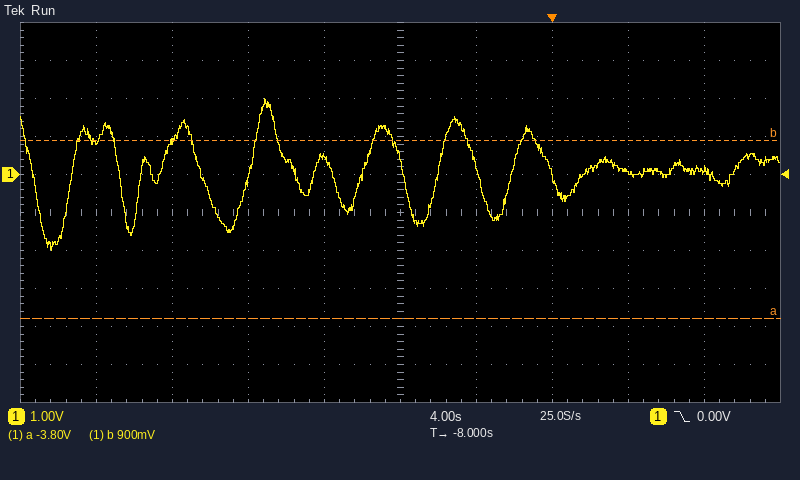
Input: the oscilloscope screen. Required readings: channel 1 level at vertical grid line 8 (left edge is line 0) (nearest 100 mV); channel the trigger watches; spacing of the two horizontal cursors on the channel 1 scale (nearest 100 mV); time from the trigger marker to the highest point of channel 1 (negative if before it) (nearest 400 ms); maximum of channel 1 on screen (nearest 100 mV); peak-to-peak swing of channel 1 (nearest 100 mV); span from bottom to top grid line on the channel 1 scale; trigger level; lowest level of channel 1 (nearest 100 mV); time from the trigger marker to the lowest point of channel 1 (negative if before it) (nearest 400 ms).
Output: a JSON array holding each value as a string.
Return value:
["100 mV", "channel 1", "4.7 V", "-15.2 s", "2.0 V", "4.0 V", "10 V", "0.00 V", "-2.0 V", "-26.4 s"]
